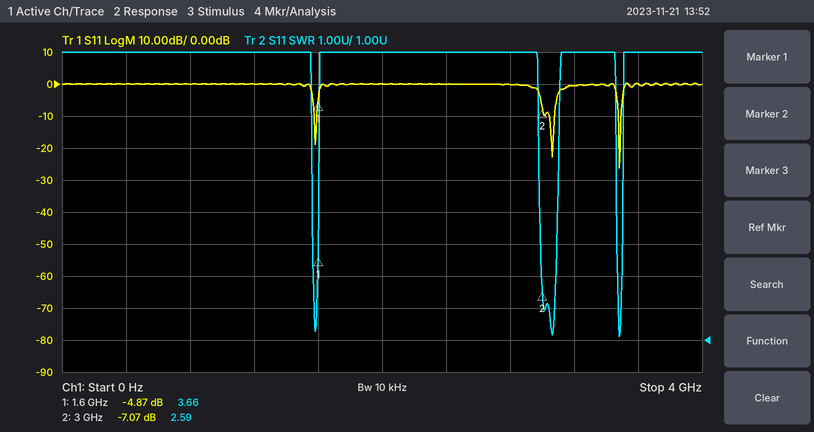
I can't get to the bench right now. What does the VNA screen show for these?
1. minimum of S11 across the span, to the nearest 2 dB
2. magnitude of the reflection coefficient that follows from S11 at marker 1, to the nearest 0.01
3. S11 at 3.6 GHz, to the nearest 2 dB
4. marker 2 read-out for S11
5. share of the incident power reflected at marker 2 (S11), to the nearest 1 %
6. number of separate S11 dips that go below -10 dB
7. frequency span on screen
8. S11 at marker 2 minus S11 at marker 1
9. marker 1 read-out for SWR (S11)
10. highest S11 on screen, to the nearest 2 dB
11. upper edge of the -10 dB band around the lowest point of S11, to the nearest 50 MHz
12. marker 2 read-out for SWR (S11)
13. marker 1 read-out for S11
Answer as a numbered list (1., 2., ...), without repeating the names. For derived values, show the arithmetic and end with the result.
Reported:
1. -26 dB
2. 10^(-4.87/20) ≈ 0.57
3. 0 dB
4. -7.07 dB
5. 10^(-7.07/10) ≈ 20 %
6. 3
7. 4 GHz
8. -7.07 − (-4.87) = -2.20 dB
9. 3.66
10. 0 dB
11. 3.50 GHz
12. 2.59
13. -4.87 dB
